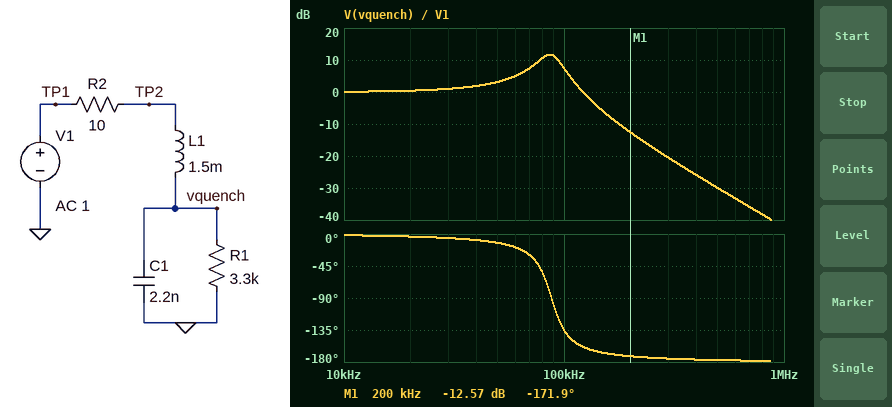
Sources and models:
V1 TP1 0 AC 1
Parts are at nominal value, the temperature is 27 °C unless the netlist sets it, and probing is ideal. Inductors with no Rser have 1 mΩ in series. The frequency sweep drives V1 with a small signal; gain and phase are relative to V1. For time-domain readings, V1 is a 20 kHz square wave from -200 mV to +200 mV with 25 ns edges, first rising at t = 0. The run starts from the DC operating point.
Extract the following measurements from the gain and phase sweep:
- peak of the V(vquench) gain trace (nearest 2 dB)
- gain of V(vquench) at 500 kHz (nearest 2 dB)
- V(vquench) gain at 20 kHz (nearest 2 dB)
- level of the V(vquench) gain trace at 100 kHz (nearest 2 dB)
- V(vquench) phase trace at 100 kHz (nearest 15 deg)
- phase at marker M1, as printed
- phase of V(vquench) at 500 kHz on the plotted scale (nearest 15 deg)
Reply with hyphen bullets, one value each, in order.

- 12 dB
- -30 dB
- 0 dB
- 8 dB
- -135 deg
- -171.9 deg
- -180 deg
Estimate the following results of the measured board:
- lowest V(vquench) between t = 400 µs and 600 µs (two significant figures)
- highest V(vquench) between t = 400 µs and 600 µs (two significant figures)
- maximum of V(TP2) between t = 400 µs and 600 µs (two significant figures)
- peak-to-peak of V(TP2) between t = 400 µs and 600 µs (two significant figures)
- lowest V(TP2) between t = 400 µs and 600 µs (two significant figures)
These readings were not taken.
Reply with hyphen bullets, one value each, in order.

- -440 mV
- 440 mV
- 200 mV
- 400 mV
- -200 mV
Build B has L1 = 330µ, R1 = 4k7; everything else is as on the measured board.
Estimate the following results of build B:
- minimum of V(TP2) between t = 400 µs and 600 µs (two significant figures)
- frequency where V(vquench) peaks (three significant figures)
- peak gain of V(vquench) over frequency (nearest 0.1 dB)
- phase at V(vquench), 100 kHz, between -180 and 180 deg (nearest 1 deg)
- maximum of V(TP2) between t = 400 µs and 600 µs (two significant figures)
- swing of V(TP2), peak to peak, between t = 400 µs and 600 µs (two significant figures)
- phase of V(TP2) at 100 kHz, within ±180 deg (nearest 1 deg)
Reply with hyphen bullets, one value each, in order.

- -210 mV
- 186 kHz
- 19.3 dB
- -5 deg
- 210 mV
- 420 mV
- -1 deg
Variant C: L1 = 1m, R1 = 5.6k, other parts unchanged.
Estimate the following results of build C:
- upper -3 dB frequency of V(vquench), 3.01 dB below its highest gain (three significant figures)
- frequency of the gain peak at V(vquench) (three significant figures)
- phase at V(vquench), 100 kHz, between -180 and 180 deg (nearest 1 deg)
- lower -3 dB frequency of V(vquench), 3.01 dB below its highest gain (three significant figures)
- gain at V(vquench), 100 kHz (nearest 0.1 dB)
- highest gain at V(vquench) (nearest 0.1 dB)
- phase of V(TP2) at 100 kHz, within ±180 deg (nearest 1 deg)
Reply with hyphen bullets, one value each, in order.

- 114 kHz
- 107 kHz
- -43 deg
- 99.4 kHz
- 14.7 dB
- 17.4 dB
- -3 deg
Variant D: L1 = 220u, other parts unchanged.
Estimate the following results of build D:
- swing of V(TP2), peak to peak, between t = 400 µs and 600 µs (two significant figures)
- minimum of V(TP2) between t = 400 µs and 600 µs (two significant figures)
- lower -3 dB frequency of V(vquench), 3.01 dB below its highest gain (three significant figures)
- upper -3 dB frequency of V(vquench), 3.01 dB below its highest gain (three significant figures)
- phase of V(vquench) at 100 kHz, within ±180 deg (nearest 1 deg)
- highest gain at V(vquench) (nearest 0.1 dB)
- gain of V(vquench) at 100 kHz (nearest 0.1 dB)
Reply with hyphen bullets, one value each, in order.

- 420 mV
- -210 mV
- 213 kHz
- 242 kHz
- -4 deg
- 17.9 dB
- 1.8 dB
